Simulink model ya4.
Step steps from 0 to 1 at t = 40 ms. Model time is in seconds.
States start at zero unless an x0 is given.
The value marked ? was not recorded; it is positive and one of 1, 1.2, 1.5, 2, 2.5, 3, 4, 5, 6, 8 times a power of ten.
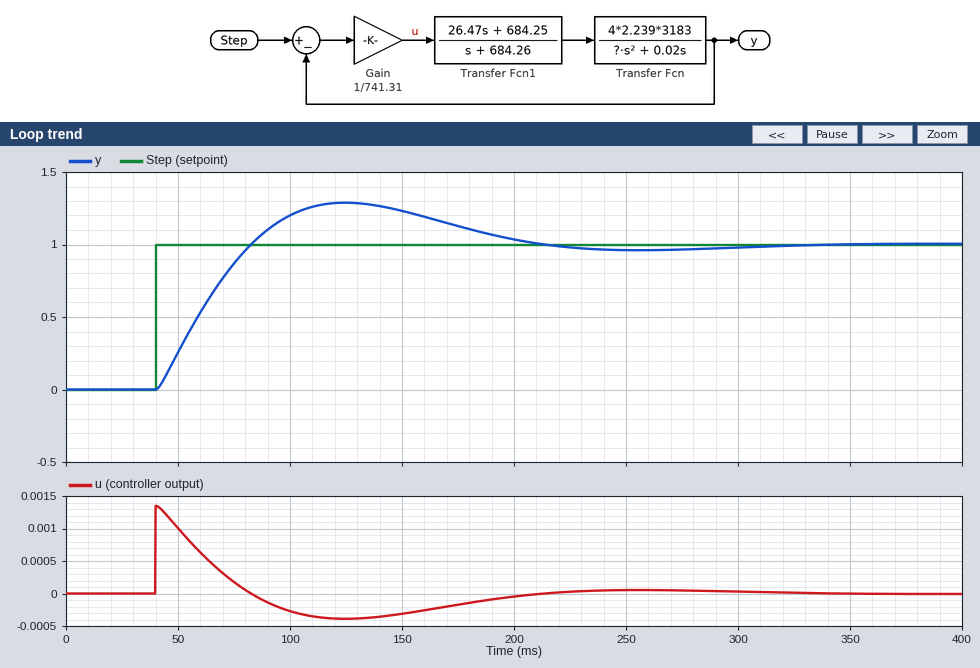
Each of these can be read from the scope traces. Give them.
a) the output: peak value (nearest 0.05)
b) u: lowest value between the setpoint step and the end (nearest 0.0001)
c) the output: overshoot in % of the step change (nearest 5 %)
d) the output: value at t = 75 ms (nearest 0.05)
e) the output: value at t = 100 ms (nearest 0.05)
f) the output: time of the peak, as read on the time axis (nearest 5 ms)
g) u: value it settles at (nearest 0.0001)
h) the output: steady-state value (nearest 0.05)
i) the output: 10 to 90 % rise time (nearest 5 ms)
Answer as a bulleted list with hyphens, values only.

- 1.30
- -0.0004
- 30 %
- 0.85
- 1.20
- 125 ms
- 0.0000
- 1.00
- 30 ms
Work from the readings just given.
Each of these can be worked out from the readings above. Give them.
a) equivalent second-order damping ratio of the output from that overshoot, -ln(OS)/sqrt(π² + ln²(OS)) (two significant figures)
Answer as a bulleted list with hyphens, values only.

- 0.36
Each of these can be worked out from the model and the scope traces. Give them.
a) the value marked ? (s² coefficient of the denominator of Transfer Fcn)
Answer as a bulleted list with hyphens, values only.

- 0.05
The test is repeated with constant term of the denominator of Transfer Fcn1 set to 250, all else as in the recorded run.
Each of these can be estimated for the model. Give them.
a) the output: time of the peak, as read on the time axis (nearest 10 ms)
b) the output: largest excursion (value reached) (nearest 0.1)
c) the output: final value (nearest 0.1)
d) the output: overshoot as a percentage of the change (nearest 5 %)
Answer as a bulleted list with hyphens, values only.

- 80 ms
- 1.2
- 1.0
- 25 %
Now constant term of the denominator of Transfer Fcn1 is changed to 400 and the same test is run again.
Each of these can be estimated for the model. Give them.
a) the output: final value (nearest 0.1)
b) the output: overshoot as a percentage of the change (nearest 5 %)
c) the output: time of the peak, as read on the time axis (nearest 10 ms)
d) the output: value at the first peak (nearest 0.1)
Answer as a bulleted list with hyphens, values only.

- 1.0
- 25 %
- 100 ms
- 1.2
